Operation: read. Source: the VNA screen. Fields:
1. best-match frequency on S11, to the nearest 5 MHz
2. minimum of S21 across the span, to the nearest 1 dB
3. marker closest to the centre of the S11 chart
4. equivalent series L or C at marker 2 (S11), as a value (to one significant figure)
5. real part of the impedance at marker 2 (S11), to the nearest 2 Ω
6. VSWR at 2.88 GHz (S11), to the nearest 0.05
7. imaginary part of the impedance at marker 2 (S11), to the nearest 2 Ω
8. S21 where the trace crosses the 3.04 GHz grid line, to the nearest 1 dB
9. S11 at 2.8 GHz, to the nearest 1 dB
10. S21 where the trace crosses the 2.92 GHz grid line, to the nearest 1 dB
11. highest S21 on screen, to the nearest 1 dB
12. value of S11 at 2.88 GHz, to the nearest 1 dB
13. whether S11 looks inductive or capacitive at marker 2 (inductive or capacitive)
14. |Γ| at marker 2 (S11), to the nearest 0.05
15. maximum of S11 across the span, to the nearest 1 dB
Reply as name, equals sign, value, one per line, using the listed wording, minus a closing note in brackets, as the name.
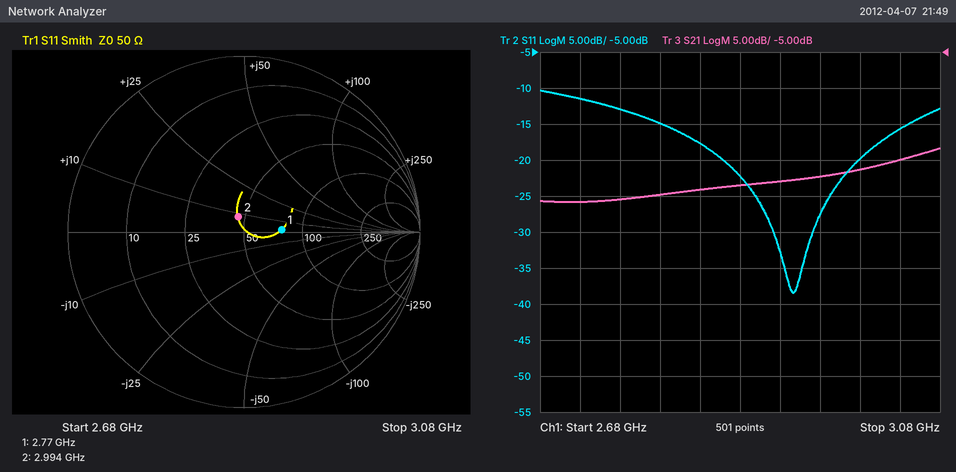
best-match frequency on S11, to the nearest 5 MHz = 2.935 GHz
minimum of S21 across the span, to the nearest 1 dB = -26 dB
marker closest to the centre of the S11 chart = marker 2
equivalent series L or C at marker 2 (S11), as a value = 400 pH
real part of the impedance at marker 2 (S11), to the nearest 2 Ω = 46 Ω
VSWR at 2.88 GHz (S11), to the nearest 0.05 = 1.15
imaginary part of the impedance at marker 2 (S11), to the nearest 2 Ω = +8 Ω
S21 where the trace crosses the 3.04 GHz grid line, to the nearest 1 dB = -20 dB
S11 at 2.8 GHz, to the nearest 1 dB = -15 dB
S21 where the trace crosses the 2.92 GHz grid line, to the nearest 1 dB = -23 dB
highest S21 on screen, to the nearest 1 dB = -18 dB
value of S11 at 2.88 GHz, to the nearest 1 dB = -22 dB
whether S11 looks inductive or capacitive at marker 2 = inductive
|Γ| at marker 2 (S11), to the nearest 0.05 = 0.10
maximum of S11 across the span, to the nearest 1 dB = -10 dB
